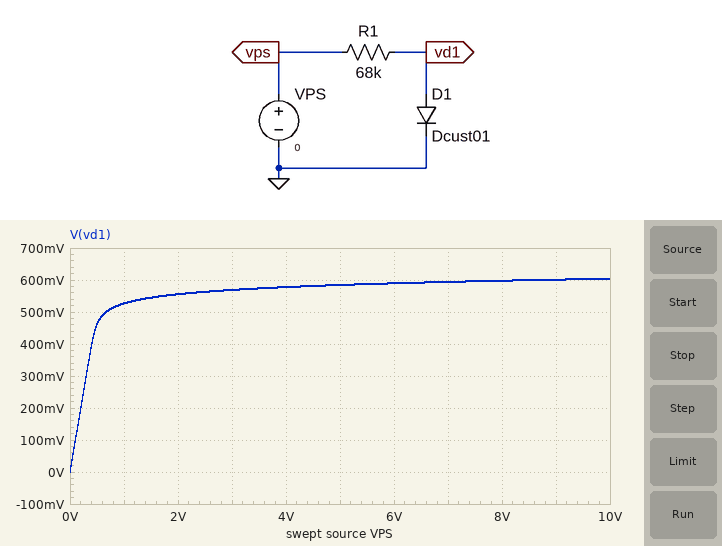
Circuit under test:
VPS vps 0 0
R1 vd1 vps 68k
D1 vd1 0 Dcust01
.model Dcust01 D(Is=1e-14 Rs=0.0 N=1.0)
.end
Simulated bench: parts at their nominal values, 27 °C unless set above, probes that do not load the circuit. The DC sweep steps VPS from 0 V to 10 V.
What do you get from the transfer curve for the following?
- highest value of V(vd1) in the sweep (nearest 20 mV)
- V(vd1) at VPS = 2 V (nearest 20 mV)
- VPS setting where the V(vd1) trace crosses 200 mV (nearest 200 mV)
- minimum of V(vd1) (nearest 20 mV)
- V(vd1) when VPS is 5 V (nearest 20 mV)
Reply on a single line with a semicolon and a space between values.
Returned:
600 mV; 560 mV; 200 mV; 0 V; 580 mV
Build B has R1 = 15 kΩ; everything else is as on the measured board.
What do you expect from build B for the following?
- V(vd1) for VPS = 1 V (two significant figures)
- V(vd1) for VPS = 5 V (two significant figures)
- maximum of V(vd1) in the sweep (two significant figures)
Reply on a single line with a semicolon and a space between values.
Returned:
560 mV; 620 mV; 640 mV
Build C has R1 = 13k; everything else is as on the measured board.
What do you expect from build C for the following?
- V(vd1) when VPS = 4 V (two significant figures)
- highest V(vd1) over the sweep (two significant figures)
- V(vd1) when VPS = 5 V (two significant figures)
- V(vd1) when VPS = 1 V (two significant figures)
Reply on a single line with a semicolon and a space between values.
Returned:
620 mV; 650 mV; 630 mV; 570 mV
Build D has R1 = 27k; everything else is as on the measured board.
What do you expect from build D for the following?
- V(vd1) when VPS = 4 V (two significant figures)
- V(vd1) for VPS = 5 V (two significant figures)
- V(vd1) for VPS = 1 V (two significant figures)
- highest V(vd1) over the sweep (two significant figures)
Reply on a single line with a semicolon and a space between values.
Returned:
600 mV; 610 mV; 550 mV; 630 mV
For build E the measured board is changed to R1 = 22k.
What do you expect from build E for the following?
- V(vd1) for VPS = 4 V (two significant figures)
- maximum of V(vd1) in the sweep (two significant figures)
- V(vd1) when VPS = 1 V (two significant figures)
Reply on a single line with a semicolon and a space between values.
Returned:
610 mV; 630 mV; 550 mV
